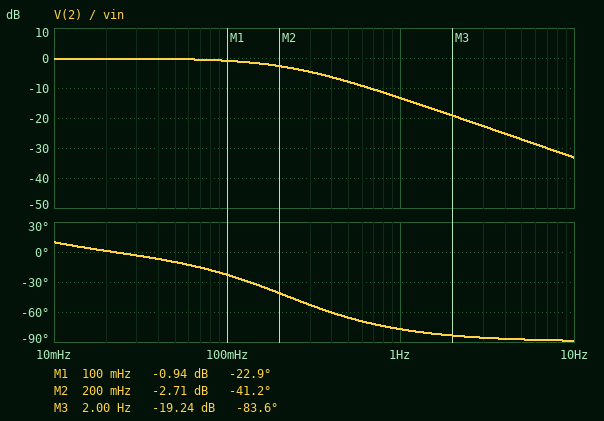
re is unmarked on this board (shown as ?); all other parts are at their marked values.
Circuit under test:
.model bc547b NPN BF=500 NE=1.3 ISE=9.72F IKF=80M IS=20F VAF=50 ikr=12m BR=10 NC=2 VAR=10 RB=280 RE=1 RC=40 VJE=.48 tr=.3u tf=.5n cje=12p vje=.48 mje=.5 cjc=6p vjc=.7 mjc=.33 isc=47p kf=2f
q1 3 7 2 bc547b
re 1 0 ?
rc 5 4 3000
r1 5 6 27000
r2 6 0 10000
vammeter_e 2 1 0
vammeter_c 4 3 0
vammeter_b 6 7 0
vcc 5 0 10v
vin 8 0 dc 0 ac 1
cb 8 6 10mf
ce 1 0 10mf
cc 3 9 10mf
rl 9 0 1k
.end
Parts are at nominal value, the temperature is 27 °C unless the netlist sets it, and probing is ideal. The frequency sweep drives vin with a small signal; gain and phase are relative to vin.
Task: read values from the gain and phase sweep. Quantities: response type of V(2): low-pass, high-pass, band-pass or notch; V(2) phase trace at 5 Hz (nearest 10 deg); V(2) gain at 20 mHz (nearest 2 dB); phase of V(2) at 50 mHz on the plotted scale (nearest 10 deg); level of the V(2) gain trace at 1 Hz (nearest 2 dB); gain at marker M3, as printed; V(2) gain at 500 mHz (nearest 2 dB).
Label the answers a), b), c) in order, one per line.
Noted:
a) low-pass
b) -90 deg
c) 0 dB
d) -10 deg
e) -14 dB
f) -19.24 dB
g) -8 dB
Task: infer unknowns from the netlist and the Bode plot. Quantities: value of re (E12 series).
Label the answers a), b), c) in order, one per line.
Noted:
a) 5.6 kΩ
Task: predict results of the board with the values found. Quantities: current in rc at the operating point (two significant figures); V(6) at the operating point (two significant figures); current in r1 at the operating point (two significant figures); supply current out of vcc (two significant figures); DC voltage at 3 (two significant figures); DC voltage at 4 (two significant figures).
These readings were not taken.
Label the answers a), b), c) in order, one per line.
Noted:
a) 370 µA
b) 2.7 V
c) 270 µA
d) 640 µA
e) 8.9 V
f) 8.9 V
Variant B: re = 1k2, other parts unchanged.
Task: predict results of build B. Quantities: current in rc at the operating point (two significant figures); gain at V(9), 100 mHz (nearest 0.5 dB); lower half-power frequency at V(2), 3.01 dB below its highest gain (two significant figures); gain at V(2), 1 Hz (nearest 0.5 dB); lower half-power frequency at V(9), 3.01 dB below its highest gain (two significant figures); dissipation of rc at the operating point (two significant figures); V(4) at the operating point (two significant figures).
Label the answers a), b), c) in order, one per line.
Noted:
a) 1.7 mA
b) 13.5 dB
c) 2.2 mHz
d) -3.5 dB
e) 890 mHz
f) 8.3 mW
g) 5.0 V
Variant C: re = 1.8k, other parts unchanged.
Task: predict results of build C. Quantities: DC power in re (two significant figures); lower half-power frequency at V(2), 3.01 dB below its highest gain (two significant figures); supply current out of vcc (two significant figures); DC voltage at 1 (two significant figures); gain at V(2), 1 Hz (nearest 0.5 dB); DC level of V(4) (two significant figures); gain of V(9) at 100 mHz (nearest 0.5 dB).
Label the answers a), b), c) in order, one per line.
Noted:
a) 2.3 mW
b) 2.2 mHz
c) 1.4 mA
d) 2.0 V
e) -5.5 dB
f) 6.6 V
g) 13.0 dB
